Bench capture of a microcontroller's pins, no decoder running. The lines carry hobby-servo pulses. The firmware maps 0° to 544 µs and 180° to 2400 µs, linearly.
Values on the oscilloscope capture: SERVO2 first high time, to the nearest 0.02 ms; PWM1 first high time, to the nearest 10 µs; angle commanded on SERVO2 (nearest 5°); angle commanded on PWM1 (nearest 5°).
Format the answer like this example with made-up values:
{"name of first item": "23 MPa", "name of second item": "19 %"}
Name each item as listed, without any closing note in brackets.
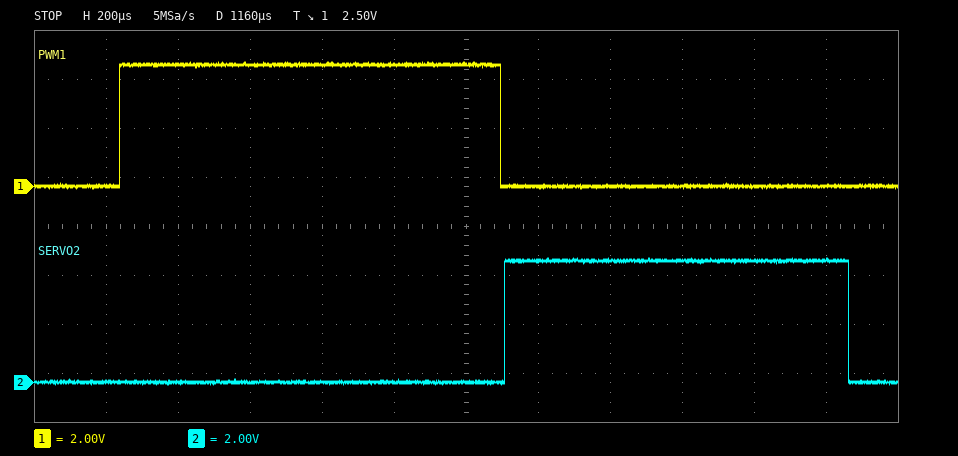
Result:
{"SERVO2 first high time, to the nearest 0.02 ms": "0.96 ms", "PWM1 first high time, to the nearest 10 µs": "1060 µs", "angle commanded on SERVO2": "40°", "angle commanded on PWM1": "50°"}
